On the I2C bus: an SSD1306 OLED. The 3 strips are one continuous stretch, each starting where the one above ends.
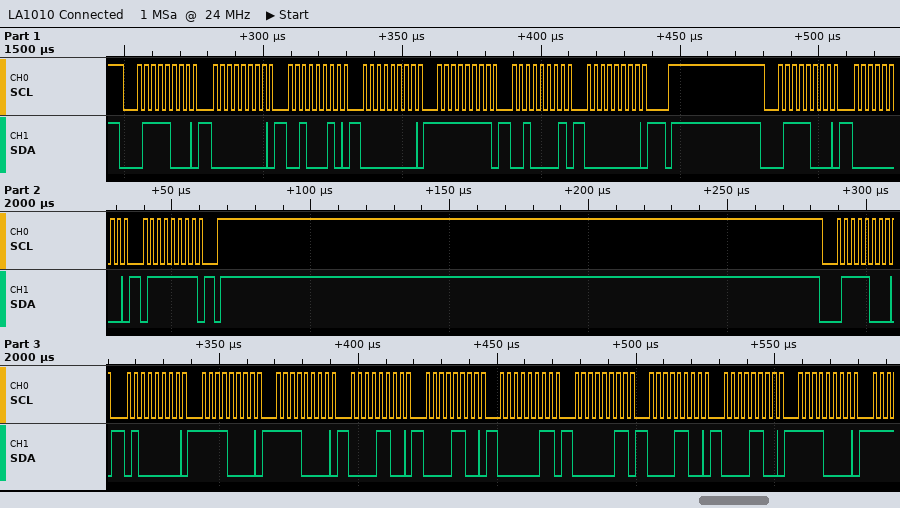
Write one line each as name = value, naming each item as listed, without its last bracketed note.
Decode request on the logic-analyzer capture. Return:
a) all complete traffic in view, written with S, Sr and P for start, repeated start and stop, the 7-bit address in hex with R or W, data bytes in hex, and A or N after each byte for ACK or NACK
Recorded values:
all complete traffic in view, written with S, Sr and P for start, repeated start and stop, the 7-bit address in hex with R or W, data bytes in hex, and A or N after each byte for ACK or NACK = S 3CW A 00 A 22 A 00 A FF A 21 A 00 A P S 3CW A 00 A 7F A P S 3CW A 40 A F0 A F0 A 0C A 0C A 03 A 03 A 0C A 0C A F0 A
